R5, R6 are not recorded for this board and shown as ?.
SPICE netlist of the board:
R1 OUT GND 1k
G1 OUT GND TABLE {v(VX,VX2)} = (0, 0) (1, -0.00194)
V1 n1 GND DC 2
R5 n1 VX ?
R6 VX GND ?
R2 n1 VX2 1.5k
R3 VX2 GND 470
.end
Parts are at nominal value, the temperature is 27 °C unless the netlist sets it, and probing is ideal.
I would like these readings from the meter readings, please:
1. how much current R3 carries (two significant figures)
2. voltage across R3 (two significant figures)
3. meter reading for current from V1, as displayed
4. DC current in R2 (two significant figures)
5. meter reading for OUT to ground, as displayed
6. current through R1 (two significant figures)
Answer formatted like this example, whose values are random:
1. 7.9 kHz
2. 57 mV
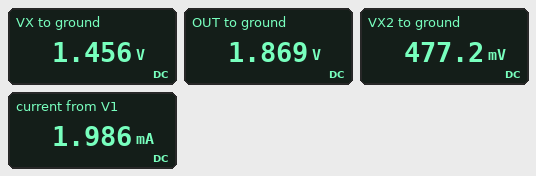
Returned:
1. 1.0 mA
2. 480 mV
3. 1.986 mA
4. 1.0 mA
5. 1.869 V
6. 1.9 mA
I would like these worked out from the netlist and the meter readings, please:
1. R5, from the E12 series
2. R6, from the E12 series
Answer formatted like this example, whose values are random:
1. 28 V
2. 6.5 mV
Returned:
1. 560 Ω
2. 1.5 kΩ
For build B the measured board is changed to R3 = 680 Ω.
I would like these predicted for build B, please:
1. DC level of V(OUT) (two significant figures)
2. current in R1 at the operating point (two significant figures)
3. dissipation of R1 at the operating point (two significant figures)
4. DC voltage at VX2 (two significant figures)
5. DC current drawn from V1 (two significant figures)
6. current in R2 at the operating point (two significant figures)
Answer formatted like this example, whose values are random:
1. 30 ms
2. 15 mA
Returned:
1. 1.6 V
2. 1.6 mA
3. 2.6 mW
4. 620 mV
5. 1.9 mA
6. 920 µA
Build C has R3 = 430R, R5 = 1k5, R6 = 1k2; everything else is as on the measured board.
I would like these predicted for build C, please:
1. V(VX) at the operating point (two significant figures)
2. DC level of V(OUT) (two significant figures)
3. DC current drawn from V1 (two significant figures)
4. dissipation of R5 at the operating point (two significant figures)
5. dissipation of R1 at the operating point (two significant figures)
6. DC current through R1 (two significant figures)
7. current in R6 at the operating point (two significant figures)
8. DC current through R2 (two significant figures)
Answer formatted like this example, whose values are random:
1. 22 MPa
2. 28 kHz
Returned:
1. 890 mV
2. 860 mV
3. 1.8 mA
4. 820 µW
5. 740 µW
6. 860 µA
7. 740 µA
8. 1.0 mA
